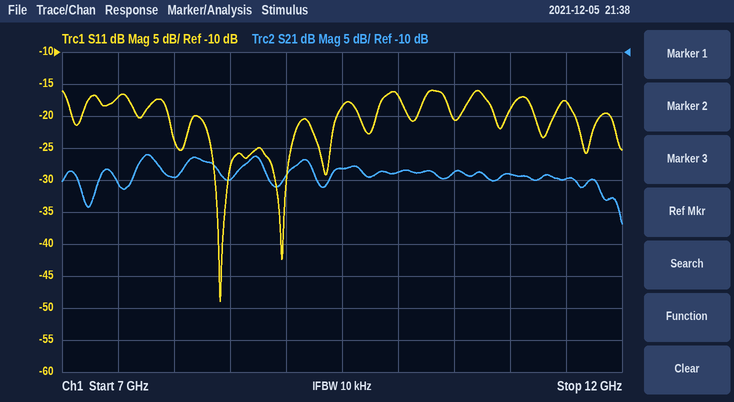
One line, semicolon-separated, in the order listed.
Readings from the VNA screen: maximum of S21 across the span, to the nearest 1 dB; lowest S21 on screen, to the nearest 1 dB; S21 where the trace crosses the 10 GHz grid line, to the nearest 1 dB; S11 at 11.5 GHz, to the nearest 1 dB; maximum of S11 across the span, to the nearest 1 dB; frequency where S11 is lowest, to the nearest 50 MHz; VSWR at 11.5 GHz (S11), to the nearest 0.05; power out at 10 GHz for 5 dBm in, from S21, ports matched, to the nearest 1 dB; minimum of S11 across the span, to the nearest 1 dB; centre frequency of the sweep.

-26 dB; -37 dB; -29 dB; -18 dB; -16 dB; 8.40 GHz; 1.30; -24 dBm; -49 dB; 9.5 GHz
